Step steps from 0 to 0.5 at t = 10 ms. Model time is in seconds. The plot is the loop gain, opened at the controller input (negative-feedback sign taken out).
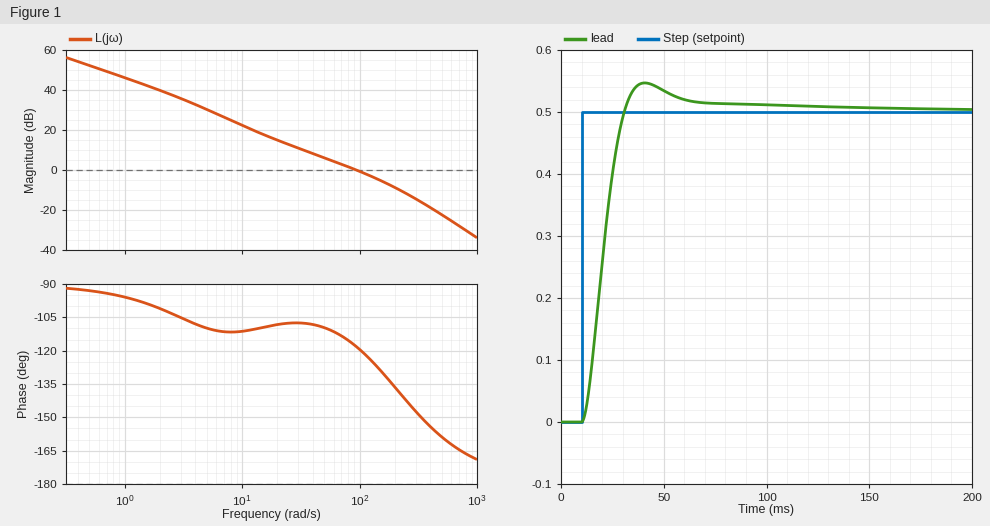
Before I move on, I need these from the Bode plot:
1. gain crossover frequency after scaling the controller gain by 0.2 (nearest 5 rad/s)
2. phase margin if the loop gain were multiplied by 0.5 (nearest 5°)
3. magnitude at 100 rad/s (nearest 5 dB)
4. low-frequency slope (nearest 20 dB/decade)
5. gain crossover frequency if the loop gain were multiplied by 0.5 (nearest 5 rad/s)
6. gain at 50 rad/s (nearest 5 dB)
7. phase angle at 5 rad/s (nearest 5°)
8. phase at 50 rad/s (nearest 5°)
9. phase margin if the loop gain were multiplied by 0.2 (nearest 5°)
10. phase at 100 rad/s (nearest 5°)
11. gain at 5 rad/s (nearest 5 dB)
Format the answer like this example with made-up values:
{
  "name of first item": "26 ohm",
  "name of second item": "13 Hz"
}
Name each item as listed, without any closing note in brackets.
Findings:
{
  "gain crossover frequency after scaling the controller gain by 0.2": "20 rad/s",
  "phase margin if the loop gain were multiplied by 0.5": "70°",
  "magnitude at 100 rad/s": "0 dB",
  "low-frequency slope": "-20 dB/decade",
  "gain crossover frequency if the loop gain were multiplied by 0.5": "50 rad/s",
  "gain at 50 rad/s": "5 dB",
  "phase angle at 5 rad/s": "-110°",
  "phase at 50 rad/s": "-110°",
  "phase margin if the loop gain were multiplied by 0.2": "70°",
  "phase at 100 rad/s": "-120°",
  "gain at 5 rad/s": "30 dB"
}
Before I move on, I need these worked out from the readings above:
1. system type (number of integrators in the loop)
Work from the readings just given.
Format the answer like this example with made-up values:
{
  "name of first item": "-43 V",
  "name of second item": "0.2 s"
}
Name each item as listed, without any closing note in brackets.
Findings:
{
  "system type": "1"
}
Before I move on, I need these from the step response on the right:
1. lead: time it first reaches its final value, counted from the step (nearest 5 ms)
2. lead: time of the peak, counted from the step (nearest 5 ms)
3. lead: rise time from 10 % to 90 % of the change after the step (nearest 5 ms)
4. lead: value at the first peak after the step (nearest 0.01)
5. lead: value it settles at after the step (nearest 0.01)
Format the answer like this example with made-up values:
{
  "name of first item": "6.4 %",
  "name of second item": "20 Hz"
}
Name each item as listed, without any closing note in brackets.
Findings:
{
  "lead: time it first reaches its final value, counted from the step": "20 ms",
  "lead: time of the peak, counted from the step": "30 ms",
  "lead: rise time from 10 % to 90 % of the change after the step": "15 ms",
  "lead: value at the first peak after the step": "0.55",
  "lead: value it settles at after the step": "0.50"
}
